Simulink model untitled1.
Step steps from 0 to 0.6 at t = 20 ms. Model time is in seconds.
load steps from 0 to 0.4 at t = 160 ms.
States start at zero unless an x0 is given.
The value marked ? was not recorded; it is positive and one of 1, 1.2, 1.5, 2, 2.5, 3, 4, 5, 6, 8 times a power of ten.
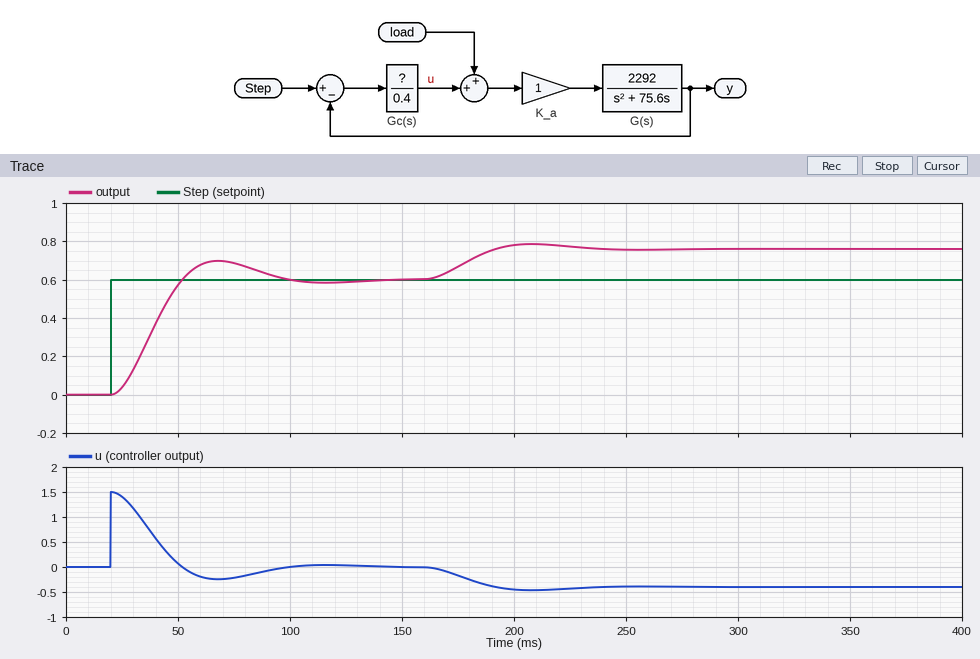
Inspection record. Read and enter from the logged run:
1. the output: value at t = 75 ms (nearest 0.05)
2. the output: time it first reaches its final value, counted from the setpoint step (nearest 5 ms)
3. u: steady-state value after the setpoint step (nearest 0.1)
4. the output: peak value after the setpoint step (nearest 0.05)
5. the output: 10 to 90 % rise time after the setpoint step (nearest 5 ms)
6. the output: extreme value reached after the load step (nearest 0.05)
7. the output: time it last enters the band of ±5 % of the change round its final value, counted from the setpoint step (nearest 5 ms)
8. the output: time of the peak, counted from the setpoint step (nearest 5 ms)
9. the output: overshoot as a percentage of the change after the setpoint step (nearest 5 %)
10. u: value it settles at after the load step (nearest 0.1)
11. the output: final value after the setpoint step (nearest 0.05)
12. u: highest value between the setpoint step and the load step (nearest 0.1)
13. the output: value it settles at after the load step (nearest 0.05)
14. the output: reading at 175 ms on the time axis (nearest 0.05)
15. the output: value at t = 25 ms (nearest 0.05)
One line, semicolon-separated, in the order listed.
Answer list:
0.70; 30 ms; 0.0; 0.70; 20 ms; 0.80; 70 ms; 50 ms; 15 %; -0.4; 0.60; 1.5; 0.75; 0.65; 0.05
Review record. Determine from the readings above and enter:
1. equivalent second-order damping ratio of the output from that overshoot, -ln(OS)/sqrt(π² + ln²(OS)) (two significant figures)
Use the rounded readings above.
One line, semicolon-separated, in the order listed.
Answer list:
0.52
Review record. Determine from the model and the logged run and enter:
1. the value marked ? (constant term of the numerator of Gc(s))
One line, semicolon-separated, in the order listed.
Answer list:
1
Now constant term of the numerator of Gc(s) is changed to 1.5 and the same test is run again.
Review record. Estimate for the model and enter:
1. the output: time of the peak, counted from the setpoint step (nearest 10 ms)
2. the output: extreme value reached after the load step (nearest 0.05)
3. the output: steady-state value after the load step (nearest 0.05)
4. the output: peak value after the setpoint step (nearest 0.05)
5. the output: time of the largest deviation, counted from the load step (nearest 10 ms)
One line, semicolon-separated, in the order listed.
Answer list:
40 ms; 0.75; 0.70; 0.75; 40 ms
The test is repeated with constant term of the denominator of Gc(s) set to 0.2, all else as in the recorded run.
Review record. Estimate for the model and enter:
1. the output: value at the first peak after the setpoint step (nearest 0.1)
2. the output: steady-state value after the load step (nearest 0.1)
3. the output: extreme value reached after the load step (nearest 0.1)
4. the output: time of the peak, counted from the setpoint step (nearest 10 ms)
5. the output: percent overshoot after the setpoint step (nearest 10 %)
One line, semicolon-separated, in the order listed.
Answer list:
0.8; 0.7; 0.7; 30 ms; 30 %
